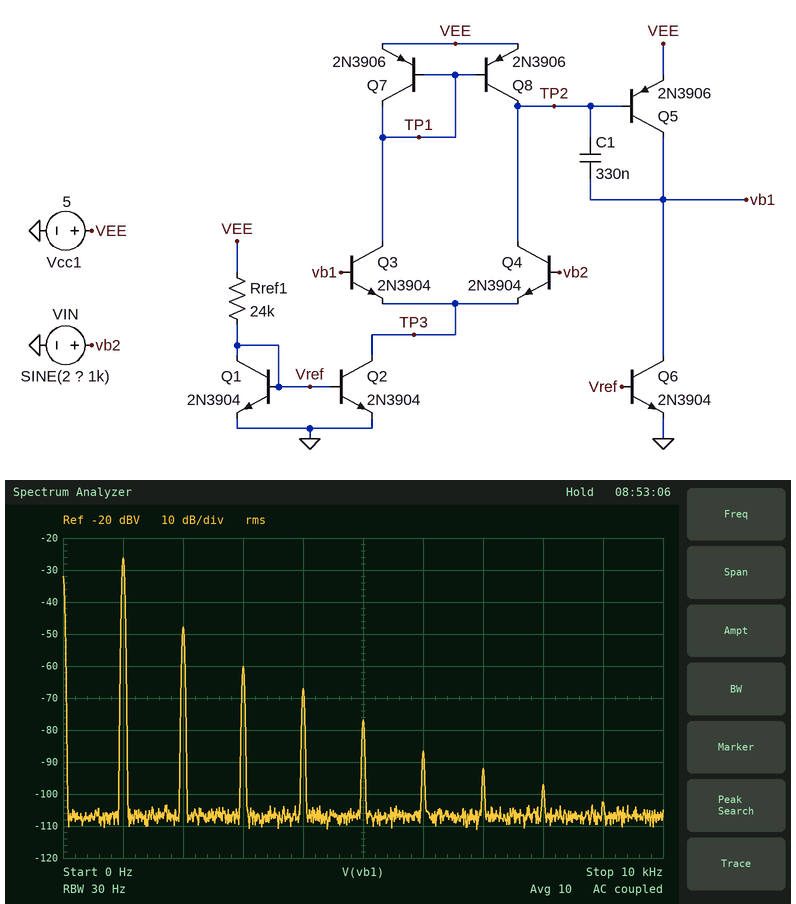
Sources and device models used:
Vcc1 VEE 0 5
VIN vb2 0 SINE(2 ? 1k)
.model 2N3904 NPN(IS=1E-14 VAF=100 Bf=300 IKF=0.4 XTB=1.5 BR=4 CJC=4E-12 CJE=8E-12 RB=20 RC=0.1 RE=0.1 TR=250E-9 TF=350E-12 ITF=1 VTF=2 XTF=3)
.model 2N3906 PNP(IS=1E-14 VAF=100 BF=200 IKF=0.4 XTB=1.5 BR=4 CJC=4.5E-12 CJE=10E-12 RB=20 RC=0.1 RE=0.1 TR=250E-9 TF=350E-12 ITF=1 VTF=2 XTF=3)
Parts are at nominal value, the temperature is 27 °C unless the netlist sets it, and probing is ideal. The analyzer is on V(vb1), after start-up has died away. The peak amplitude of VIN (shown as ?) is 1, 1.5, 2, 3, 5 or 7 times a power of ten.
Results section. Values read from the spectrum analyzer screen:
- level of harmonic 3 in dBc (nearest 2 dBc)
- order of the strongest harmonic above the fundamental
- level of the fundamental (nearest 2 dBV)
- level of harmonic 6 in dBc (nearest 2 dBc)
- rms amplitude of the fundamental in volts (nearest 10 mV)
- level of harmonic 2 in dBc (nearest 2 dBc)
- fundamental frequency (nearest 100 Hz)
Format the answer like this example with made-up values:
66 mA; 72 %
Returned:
-34 dBc; 2; -26 dBV; -60 dBc; 50 mV; -22 dBc; 1.0 kHz
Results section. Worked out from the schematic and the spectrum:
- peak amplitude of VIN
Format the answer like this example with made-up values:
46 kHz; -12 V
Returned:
70 mV
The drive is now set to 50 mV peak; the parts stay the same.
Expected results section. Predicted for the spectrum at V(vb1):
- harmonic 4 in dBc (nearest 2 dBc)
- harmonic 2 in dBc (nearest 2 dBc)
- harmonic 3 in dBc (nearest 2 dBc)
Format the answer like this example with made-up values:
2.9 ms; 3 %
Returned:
-52 dBc; -26 dBc; -42 dBc
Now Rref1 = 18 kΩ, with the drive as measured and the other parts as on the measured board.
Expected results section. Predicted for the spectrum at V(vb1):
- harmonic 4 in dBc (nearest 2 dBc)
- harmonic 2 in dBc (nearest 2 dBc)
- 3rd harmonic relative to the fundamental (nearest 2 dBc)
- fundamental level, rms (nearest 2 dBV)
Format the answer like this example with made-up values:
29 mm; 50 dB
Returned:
-50 dBc; -30 dBc; -42 dBc; -26 dBV
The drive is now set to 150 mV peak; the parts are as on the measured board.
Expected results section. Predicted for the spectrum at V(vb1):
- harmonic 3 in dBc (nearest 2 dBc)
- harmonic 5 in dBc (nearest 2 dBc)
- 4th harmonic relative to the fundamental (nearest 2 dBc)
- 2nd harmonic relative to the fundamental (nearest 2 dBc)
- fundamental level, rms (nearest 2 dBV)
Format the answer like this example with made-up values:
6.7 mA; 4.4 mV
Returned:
-18 dBc; -30 dBc; -22 dBc; -18 dBc; -22 dBV
